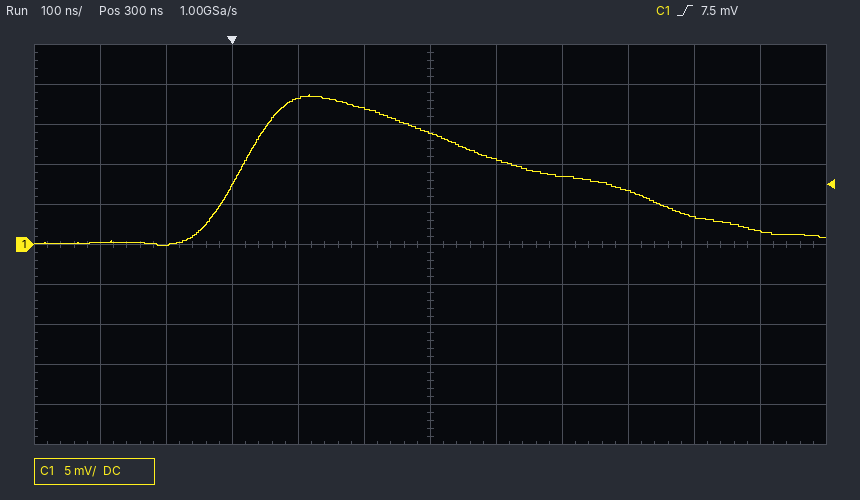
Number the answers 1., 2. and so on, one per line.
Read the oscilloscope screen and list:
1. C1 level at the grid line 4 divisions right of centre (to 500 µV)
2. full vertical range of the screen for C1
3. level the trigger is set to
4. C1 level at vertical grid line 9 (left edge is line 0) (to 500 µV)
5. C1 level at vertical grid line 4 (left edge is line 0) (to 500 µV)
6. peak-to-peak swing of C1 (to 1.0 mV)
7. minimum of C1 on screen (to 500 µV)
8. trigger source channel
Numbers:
1. 3.5 mV
2. 50 mV
3. 7.5 mV
4. 6.5 mV
5. 18.5 mV
6. 19.0 mV
7. 0.0 mV
8. C1
